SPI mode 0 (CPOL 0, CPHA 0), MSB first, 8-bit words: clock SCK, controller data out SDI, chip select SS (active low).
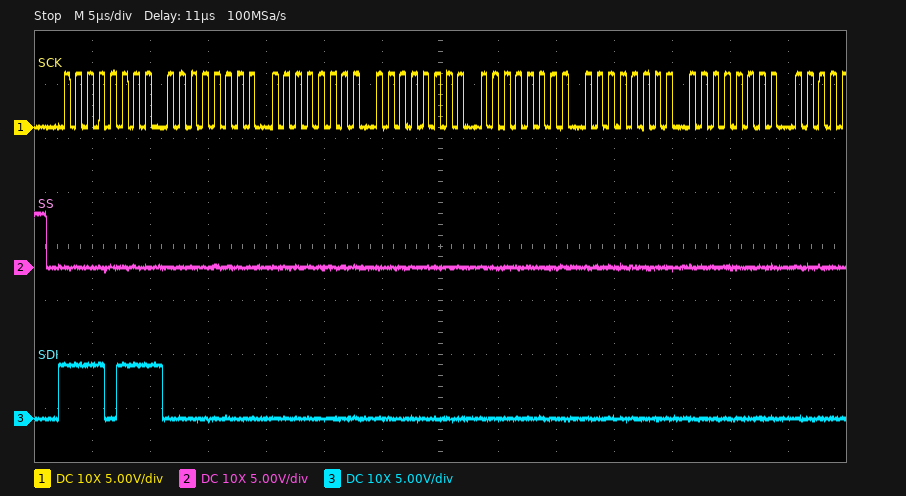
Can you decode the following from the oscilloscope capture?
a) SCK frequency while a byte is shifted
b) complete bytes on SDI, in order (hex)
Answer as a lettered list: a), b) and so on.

a) 1 MHz
b) 0xF7 0x00 0x00 0x00 0x00 0x00 0x00
